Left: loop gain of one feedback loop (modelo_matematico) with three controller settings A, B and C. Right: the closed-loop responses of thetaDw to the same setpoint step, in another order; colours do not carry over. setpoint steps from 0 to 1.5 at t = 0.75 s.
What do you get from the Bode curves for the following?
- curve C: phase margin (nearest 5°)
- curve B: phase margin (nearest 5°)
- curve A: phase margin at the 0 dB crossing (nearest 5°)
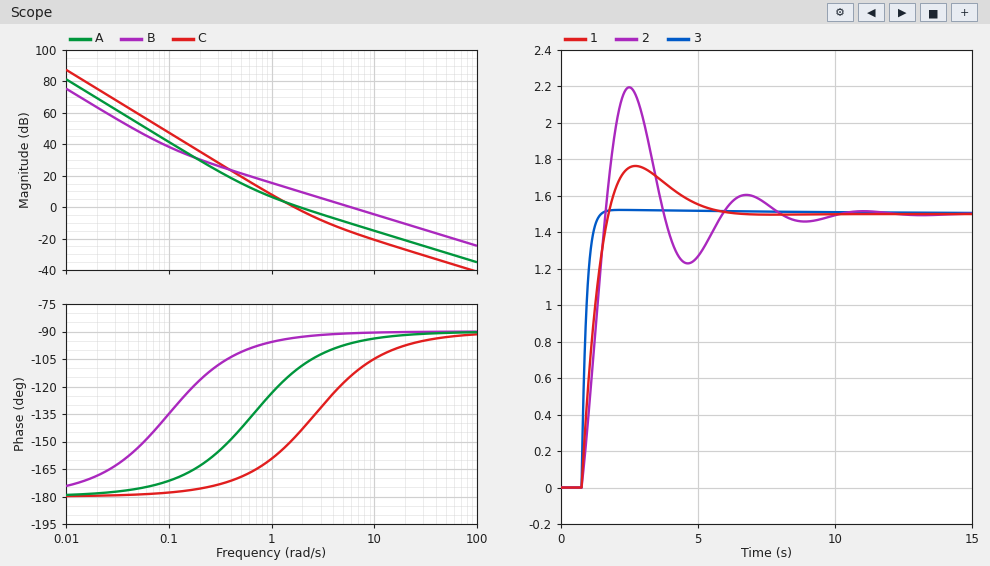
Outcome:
30°
90°
70°
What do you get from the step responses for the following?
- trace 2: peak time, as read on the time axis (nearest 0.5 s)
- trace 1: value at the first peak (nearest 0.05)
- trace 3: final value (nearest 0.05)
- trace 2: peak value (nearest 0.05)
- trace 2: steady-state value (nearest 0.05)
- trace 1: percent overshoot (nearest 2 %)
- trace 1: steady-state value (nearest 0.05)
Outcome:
2.5 s
1.75
1.50
2.20
1.50
18 %
1.50
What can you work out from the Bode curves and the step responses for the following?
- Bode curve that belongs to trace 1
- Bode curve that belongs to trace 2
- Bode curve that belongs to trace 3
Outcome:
A
C
B
